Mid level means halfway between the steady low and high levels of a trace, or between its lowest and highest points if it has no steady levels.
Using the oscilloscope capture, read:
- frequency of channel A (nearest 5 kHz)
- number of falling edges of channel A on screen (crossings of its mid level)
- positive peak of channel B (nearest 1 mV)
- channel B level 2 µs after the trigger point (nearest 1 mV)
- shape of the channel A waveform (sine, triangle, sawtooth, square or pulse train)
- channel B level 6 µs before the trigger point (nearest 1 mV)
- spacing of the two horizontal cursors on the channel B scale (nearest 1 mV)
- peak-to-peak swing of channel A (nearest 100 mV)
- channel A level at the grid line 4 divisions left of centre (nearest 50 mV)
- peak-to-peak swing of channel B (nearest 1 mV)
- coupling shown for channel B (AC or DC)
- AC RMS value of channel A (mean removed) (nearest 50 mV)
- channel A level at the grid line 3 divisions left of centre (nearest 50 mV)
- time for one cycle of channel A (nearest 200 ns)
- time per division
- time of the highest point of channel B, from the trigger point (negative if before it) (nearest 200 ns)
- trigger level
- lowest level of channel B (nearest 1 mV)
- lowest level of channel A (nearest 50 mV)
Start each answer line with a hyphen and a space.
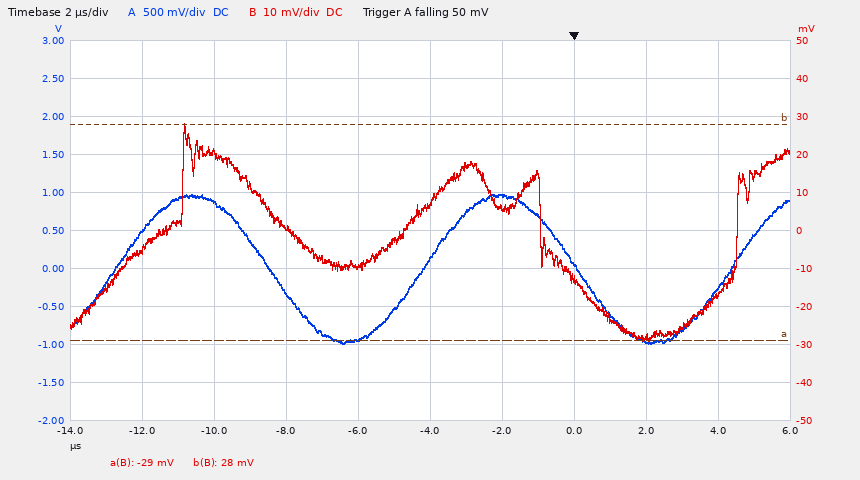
- 115 kHz
- 2
- 28 mV
- -28 mV
- sine
- -9 mV
- 57 mV
- 2.00 V
- 500 mV
- 57 mV
- DC
- 700 mV
- 850 mV
- 8.6 µs
- 2 µs
- -10.8 µs
- 50 mV
- -29 mV
- -1.00 V
